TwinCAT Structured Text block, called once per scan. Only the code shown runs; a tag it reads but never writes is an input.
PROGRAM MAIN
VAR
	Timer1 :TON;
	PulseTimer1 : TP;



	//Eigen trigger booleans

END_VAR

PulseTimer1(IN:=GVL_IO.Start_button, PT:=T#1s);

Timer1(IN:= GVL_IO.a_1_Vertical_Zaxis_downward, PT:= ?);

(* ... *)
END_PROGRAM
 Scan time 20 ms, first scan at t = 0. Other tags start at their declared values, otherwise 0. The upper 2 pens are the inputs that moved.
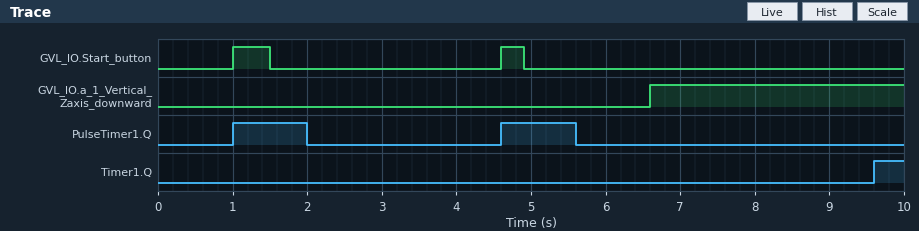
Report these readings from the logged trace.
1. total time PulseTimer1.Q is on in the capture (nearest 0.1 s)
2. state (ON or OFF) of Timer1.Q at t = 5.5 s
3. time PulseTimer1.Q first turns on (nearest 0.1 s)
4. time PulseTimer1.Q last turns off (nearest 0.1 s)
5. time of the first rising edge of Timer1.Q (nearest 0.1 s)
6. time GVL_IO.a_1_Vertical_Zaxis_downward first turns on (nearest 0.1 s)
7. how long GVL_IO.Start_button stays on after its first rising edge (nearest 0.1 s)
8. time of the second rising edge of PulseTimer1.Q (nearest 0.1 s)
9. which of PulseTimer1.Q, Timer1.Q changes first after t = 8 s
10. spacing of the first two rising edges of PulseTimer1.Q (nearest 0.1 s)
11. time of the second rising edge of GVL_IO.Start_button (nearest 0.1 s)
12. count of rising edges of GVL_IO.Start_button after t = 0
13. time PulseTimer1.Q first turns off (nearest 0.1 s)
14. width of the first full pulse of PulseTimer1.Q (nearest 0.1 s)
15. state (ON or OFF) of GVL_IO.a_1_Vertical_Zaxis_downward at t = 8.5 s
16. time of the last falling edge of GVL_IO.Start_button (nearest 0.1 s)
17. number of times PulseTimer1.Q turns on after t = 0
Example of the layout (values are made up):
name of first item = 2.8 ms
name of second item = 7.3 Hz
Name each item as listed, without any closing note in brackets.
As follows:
total time PulseTimer1.Q is on in the capture = 2.0 s
state (ON or OFF) of Timer1.Q at t = 5.5 s = OFF
time PulseTimer1.Q first turns on = 1.0 s
time PulseTimer1.Q last turns off = 5.6 s
time of the first rising edge of Timer1.Q = 9.6 s
time GVL_IO.a_1_Vertical_Zaxis_downward first turns on = 6.6 s
how long GVL_IO.Start_button stays on after its first rising edge = 0.5 s
time of the second rising edge of PulseTimer1.Q = 4.6 s
which of PulseTimer1.Q, Timer1.Q changes first after t = 8 s = Timer1.Q
spacing of the first two rising edges of PulseTimer1.Q = 3.6 s
time of the second rising edge of GVL_IO.Start_button = 4.6 s
count of rising edges of GVL_IO.Start_button after t = 0 = 2
time PulseTimer1.Q first turns off = 2.0 s
width of the first full pulse of PulseTimer1.Q = 1.0 s
state (ON or OFF) of GVL_IO.a_1_Vertical_Zaxis_downward at t = 8.5 s = ON
time of the last falling edge of GVL_IO.Start_button = 4.9 s
number of times PulseTimer1.Q turns on after t = 0 = 2
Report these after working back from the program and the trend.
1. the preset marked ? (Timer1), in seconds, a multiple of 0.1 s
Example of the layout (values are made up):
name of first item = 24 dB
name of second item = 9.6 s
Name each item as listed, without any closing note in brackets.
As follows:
the preset marked ? (Timer1), in seconds, a multiple of 0.1 s = 3.0 s
